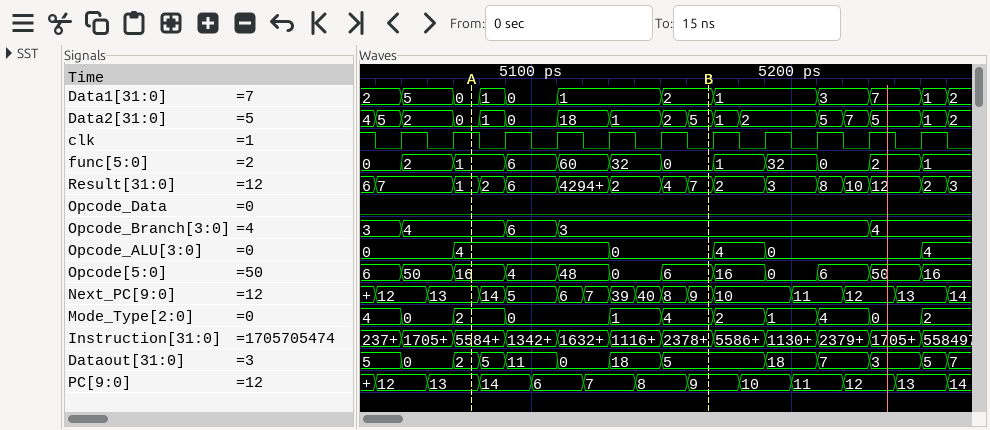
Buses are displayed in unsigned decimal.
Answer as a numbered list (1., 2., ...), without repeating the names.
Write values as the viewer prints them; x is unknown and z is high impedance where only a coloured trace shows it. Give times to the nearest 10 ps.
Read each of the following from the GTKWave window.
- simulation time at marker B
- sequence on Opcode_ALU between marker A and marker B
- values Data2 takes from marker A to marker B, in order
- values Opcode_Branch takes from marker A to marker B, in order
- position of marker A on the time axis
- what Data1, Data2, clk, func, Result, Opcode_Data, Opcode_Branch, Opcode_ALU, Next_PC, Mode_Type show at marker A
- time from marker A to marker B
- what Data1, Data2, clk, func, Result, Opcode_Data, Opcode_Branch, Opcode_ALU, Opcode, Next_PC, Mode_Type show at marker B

1. 5170 ps
2. 4, 0
3. 0, 1, 0, 18, 1, 2, 5
4. 4, 6, 3
5. 5080 ps
6. Data1=0, Data2=0, clk=1, func=1, Result=1, Opcode_Data=0, Opcode_Branch=4, Opcode_ALU=4, Next_PC=13, Mode_Type=2
7. 90 ps
8. Data1=2, Data2=5, clk=0, func=0, Result=7, Opcode_Data=0, Opcode_Branch=3, Opcode_ALU=0, Opcode=6, Next_PC=9, Mode_Type=4
